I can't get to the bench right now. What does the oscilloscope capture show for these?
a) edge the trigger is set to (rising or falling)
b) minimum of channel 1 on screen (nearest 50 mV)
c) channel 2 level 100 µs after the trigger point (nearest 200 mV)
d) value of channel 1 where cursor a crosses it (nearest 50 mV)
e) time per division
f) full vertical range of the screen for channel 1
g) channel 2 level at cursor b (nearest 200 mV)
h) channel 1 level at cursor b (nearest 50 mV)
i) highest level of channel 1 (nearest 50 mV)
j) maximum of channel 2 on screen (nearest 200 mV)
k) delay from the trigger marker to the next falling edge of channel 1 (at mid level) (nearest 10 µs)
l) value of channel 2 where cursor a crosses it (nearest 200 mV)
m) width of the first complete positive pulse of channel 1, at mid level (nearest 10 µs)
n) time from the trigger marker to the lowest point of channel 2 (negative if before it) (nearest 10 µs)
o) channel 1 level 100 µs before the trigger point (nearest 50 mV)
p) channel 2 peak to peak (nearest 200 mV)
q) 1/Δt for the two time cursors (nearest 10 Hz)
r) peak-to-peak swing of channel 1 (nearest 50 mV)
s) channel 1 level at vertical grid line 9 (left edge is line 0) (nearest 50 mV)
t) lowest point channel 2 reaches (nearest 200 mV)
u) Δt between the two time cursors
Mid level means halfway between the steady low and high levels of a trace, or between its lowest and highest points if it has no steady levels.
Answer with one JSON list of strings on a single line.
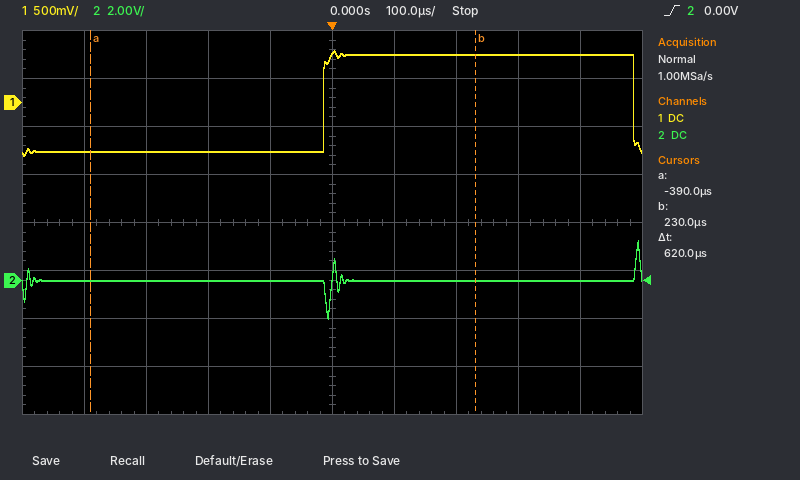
["rising", "-550 mV", "0.0 V", "-500 mV", "100 µs", "4 V", "0.0 V", "500 mV", "550 mV", "1.6 V", "490 µs", "0.0 V", "500 µs", "-10 µs", "-500 mV", "3.2 V", "1.61 kHz", "1.10 V", "500 mV", "-1.6 V", "620 µs"]
